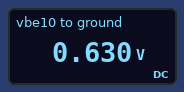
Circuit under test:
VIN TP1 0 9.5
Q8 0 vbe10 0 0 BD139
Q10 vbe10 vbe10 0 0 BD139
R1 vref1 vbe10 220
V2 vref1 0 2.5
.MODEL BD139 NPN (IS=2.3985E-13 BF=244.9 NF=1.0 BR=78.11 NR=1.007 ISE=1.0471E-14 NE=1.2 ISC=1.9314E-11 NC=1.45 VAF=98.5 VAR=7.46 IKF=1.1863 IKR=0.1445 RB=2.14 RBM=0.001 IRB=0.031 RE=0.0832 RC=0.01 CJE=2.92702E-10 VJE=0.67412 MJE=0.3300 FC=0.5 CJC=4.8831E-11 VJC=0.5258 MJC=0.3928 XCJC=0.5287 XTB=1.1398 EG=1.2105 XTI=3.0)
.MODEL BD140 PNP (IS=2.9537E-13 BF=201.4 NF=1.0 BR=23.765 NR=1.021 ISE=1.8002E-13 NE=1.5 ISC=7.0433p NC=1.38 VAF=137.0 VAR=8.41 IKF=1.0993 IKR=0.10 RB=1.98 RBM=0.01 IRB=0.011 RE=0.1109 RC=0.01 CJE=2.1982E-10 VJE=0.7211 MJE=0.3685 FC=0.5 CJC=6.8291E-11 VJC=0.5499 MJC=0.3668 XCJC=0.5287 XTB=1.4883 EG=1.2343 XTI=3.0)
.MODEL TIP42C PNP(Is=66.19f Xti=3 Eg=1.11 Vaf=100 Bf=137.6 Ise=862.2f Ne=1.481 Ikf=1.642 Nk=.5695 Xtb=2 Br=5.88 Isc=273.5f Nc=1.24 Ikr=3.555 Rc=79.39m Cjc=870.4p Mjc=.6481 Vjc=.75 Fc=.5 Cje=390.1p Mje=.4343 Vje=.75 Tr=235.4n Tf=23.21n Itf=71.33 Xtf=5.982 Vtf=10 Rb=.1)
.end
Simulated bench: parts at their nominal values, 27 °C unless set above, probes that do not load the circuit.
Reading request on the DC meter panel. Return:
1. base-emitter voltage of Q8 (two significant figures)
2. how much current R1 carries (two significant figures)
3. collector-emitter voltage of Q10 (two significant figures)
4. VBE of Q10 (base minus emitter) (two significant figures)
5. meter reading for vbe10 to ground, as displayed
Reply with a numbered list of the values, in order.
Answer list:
1. 630 mV
2. 8.5 mA
3. 630 mV
4. 630 mV
5. 0.630 V
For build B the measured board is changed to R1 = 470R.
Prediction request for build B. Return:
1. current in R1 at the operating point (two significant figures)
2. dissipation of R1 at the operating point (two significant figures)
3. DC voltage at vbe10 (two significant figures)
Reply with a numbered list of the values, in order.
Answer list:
1. 4.0 mA
2. 7.6 mW
3. 610 mV
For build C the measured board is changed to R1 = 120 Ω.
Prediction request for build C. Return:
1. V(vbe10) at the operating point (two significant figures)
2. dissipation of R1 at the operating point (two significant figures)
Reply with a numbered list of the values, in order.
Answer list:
1. 650 mV
2. 29 mW
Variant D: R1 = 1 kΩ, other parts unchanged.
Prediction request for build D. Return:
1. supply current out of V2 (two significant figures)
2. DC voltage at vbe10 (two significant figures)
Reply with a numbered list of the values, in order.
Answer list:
1. 1.9 mA
2. 590 mV
